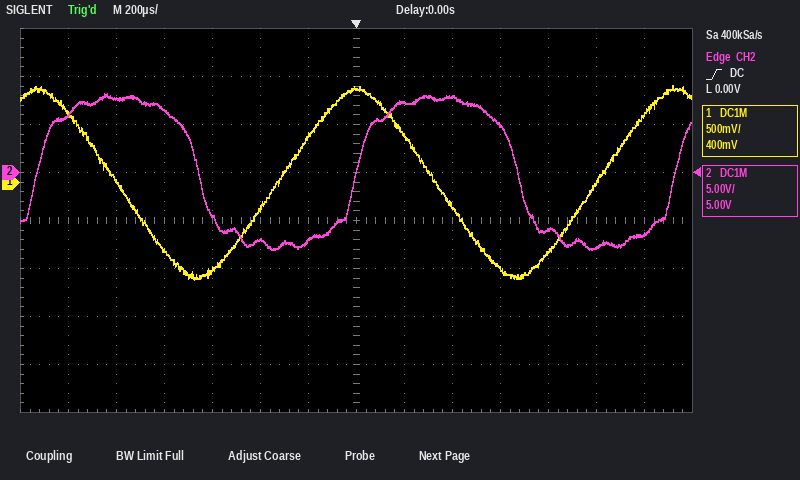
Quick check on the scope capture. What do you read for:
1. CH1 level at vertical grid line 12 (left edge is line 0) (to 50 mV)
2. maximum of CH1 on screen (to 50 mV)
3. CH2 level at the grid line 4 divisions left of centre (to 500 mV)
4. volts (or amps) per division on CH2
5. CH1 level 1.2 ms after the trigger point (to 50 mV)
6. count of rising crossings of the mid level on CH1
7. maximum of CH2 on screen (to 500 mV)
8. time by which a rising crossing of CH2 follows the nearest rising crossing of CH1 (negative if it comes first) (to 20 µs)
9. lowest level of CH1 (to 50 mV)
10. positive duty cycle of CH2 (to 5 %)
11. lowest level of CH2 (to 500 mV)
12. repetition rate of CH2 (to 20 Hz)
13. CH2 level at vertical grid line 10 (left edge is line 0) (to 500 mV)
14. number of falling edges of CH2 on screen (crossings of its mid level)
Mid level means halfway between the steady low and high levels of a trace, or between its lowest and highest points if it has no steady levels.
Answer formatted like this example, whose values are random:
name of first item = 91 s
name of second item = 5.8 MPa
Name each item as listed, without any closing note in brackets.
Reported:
CH1 level at vertical grid line 12 (left edge is line 0) = 0 mV
maximum of CH1 on screen = 1.00 V
CH2 level at the grid line 4 divisions left of centre = 6.5 V
volts (or amps) per division on CH2 = 5 V
CH1 level 1.2 ms after the trigger point = 700 mV
count of rising crossings of the mid level on CH1 = 2
maximum of CH2 on screen = 8.0 V
time by which a rising crossing of CH2 follows the nearest rising crossing of CH1 (negative if it comes first) = +320 µs
lowest level of CH1 = -1.00 V
positive duty cycle of CH2 = 50 %
lowest level of CH2 = -8.0 V
repetition rate of CH2 = 760 Hz
CH2 level at vertical grid line 10 (left edge is line 0) = 5.0 V
number of falling edges of CH2 on screen = 2
